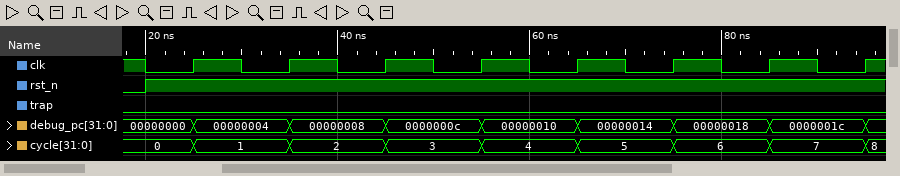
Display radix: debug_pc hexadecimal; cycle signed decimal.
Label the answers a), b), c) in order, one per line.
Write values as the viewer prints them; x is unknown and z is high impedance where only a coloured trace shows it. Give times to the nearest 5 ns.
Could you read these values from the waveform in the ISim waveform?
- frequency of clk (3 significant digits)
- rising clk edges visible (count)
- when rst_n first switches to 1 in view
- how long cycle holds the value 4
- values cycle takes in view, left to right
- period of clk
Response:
a) 100 MHz
b) 8
c) 20 ns
d) 10 ns
e) 0, 1, 2, 3, 4, 5, 6, 7, 8
f) 10 ns
